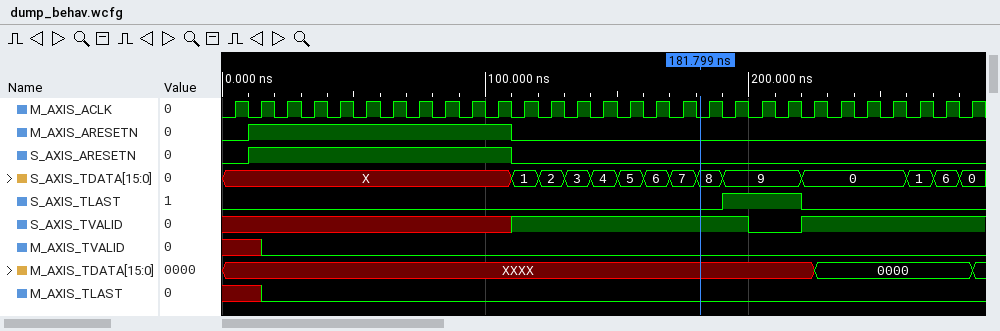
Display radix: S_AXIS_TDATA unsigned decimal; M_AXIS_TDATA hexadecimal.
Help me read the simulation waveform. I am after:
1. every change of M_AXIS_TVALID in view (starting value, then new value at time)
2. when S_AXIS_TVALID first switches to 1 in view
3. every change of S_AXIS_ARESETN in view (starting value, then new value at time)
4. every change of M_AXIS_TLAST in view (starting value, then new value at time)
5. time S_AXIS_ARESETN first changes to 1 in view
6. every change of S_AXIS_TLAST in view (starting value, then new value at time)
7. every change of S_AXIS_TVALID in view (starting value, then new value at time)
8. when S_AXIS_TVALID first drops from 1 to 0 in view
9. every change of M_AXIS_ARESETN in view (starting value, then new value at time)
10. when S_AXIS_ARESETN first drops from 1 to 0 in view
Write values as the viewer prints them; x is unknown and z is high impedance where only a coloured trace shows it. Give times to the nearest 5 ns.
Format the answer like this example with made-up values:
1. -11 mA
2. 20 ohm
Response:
1. x, 0 at 15 ns
2. 110 ns
3. 0, 1 at 10 ns, 0 at 110 ns
4. x, 0 at 15 ns
5. 10 ns
6. 0, 1 at 190 ns, 0 at 220 ns
7. x, 1 at 110 ns, 0 at 200 ns, 1 at 220 ns
8. 200 ns
9. 0, 1 at 10 ns, 0 at 110 ns
10. 110 ns
